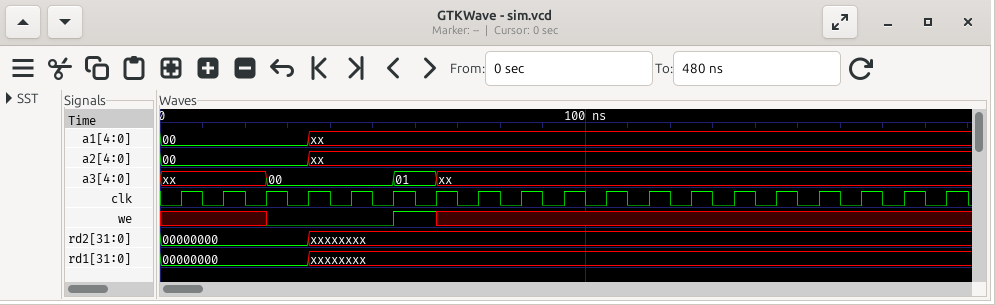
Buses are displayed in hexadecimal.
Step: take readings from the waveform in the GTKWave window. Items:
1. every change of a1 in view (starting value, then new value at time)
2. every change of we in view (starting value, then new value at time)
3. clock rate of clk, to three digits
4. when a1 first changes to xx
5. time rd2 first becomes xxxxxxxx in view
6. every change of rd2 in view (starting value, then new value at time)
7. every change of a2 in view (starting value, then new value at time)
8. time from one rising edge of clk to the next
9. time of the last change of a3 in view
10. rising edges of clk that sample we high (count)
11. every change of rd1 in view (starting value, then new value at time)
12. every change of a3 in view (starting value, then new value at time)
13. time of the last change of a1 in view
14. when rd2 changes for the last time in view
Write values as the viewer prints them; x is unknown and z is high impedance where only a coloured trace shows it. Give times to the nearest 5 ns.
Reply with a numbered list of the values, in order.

1. 00, xx at 35 ns
2. x, 0 at 25 ns, 1 at 55 ns, x at 65 ns
3. 100 MHz
4. 35 ns
5. 35 ns
6. 00000000, xxxxxxxx at 35 ns
7. 00, xx at 35 ns
8. 10 ns
9. 65 ns
10. 1
11. 00000000, xxxxxxxx at 35 ns
12. xx, 00 at 25 ns, 01 at 55 ns, xx at 65 ns
13. 35 ns
14. 35 ns
